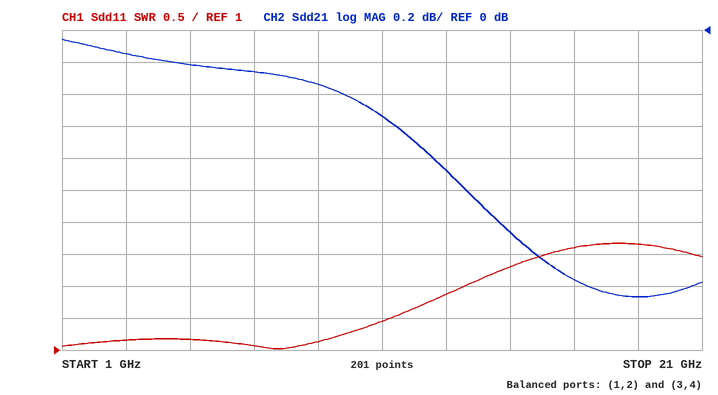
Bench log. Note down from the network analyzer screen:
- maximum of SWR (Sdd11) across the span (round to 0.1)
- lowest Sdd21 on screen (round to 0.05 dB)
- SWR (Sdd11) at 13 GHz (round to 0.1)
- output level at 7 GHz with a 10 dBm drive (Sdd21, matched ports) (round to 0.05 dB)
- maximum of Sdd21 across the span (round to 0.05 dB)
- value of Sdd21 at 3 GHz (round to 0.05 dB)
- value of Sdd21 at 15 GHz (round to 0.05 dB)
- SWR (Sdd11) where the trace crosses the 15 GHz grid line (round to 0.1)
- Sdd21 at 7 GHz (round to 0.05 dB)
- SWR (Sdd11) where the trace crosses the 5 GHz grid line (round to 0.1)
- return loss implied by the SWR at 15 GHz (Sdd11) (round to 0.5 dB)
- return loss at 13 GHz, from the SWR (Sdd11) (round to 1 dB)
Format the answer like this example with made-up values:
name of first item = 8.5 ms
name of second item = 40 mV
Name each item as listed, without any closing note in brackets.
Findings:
maximum of SWR (Sdd11) across the span = 2.7
lowest Sdd21 on screen = -1.65 dB
SWR (Sdd11) at 13 GHz = 1.9
output level at 7 GHz with a 10 dBm drive (Sdd21, matched ports) = 9.75 dBm
maximum of Sdd21 across the span = -0.05 dB
value of Sdd21 at 3 GHz = -0.15 dB
value of Sdd21 at 15 GHz = -1.25 dB
SWR (Sdd11) where the trace crosses the 15 GHz grid line = 2.3
Sdd21 at 7 GHz = -0.25 dB
SWR (Sdd11) where the trace crosses the 5 GHz grid line = 1.2
return loss implied by the SWR at 15 GHz (Sdd11) = 8.0 dB
return loss at 13 GHz, from the SWR (Sdd11) = 10 dB
